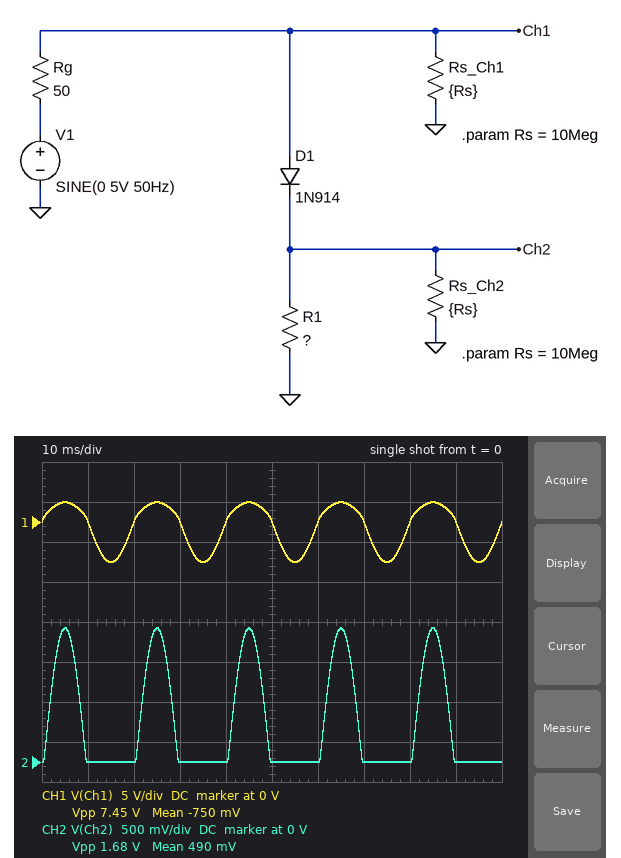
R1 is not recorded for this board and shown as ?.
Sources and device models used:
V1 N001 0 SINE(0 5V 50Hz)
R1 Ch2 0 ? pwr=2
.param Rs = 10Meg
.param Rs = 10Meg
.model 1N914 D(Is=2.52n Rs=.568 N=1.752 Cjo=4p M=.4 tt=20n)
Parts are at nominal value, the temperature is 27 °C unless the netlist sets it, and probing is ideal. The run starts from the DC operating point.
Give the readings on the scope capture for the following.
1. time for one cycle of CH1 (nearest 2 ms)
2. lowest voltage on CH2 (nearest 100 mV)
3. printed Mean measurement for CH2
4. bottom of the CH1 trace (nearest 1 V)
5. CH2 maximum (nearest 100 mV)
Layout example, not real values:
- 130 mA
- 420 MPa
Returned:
- 20 ms
- 0 V
- 490 mV
- -5 V
- 1.7 V
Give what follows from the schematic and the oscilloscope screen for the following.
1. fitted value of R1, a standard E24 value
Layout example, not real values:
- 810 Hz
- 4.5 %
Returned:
- 33 Ω
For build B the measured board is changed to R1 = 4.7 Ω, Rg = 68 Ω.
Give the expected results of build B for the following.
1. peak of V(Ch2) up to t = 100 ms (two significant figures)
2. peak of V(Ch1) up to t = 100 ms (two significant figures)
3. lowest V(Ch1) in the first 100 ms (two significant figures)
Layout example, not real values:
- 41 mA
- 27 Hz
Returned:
- 270 mV
- 1.1 V
- -5.0 V
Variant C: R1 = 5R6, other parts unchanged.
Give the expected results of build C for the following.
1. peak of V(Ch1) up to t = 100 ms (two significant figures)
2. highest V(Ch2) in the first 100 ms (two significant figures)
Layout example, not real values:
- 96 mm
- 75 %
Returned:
- 1.2 V
- 420 mV
